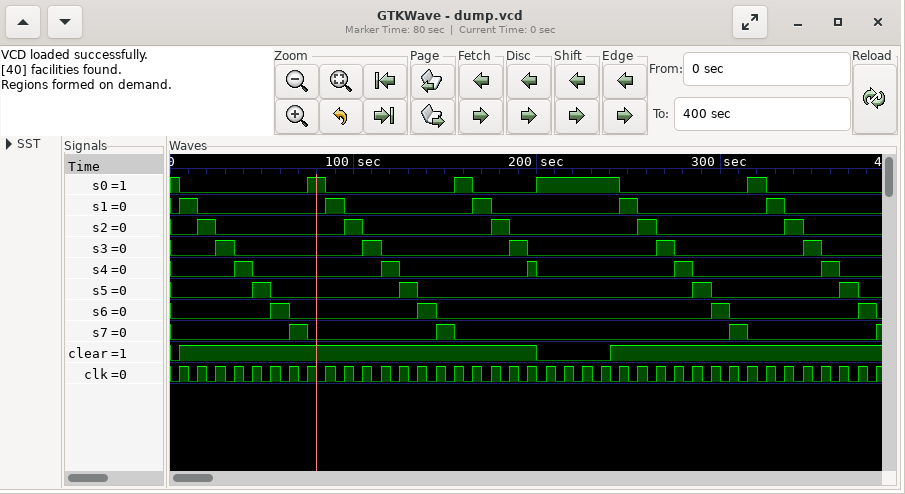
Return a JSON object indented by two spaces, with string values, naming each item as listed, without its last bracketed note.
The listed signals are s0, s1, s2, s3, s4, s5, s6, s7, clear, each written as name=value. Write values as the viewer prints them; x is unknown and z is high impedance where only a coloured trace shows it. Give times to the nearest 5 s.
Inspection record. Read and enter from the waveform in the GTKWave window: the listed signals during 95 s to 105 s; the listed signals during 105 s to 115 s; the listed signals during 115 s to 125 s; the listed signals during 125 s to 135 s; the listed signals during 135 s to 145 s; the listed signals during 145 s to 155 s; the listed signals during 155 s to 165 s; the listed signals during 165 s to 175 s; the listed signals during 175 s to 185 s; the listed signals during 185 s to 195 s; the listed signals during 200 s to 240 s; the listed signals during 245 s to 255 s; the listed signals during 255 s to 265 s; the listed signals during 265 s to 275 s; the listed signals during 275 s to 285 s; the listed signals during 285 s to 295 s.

{
  "the listed signals during 95 s to 105 s": "s0=0, s1=0, s2=1, s3=0, s4=0, s5=0, s6=0, s7=0, clear=1",
  "the listed signals during 105 s to 115 s": "s0=0, s1=0, s2=0, s3=1, s4=0, s5=0, s6=0, s7=0, clear=1",
  "the listed signals during 115 s to 125 s": "s0=0, s1=0, s2=0, s3=0, s4=1, s5=0, s6=0, s7=0, clear=1",
  "the listed signals during 125 s to 135 s": "s0=0, s1=0, s2=0, s3=0, s4=0, s5=1, s6=0, s7=0, clear=1",
  "the listed signals during 135 s to 145 s": "s0=0, s1=0, s2=0, s3=0, s4=0, s5=0, s6=1, s7=0, clear=1",
  "the listed signals during 145 s to 155 s": "s0=0, s1=0, s2=0, s3=0, s4=0, s5=0, s6=0, s7=1, clear=1",
  "the listed signals during 155 s to 165 s": "s0=1, s1=0, s2=0, s3=0, s4=0, s5=0, s6=0, s7=0, clear=1",
  "the listed signals during 165 s to 175 s": "s0=0, s1=1, s2=0, s3=0, s4=0, s5=0, s6=0, s7=0, clear=1",
  "the listed signals during 175 s to 185 s": "s0=0, s1=0, s2=1, s3=0, s4=0, s5=0, s6=0, s7=0, clear=1",
  "the listed signals during 185 s to 195 s": "s0=0, s1=0, s2=0, s3=1, s4=0, s5=0, s6=0, s7=0, clear=1",
  "the listed signals during 200 s to 240 s": "s0=1, s1=0, s2=0, s3=0, s4=0, s5=0, s6=0, s7=0, clear=0",
  "the listed signals during 245 s to 255 s": "s0=0, s1=1, s2=0, s3=0, s4=0, s5=0, s6=0, s7=0, clear=1",
  "the listed signals during 255 s to 265 s": "s0=0, s1=0, s2=1, s3=0, s4=0, s5=0, s6=0, s7=0, clear=1",
  "the listed signals during 265 s to 275 s": "s0=0, s1=0, s2=0, s3=1, s4=0, s5=0, s6=0, s7=0, clear=1",
  "the listed signals during 275 s to 285 s": "s0=0, s1=0, s2=0, s3=0, s4=1, s5=0, s6=0, s7=0, clear=1",
  "the listed signals during 285 s to 295 s": "s0=0, s1=0, s2=0, s3=0, s4=0, s5=1, s6=0, s7=0, clear=1"
}
